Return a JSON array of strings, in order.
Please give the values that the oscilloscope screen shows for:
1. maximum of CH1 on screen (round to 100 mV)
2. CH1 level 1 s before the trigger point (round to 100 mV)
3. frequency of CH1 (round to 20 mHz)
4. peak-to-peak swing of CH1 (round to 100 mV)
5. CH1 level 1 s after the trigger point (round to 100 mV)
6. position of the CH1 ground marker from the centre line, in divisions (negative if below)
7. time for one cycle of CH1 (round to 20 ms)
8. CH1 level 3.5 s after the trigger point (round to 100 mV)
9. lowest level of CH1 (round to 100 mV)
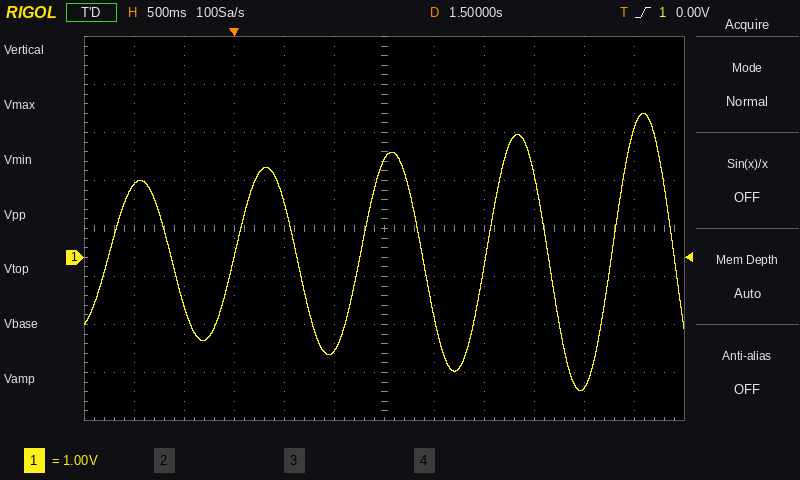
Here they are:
["3.0 V", "1.5 V", "800 mHz", "5.8 V", "-1.9 V", "-0.6 div", "1.26 s", "-2.7 V", "-2.8 V"]
